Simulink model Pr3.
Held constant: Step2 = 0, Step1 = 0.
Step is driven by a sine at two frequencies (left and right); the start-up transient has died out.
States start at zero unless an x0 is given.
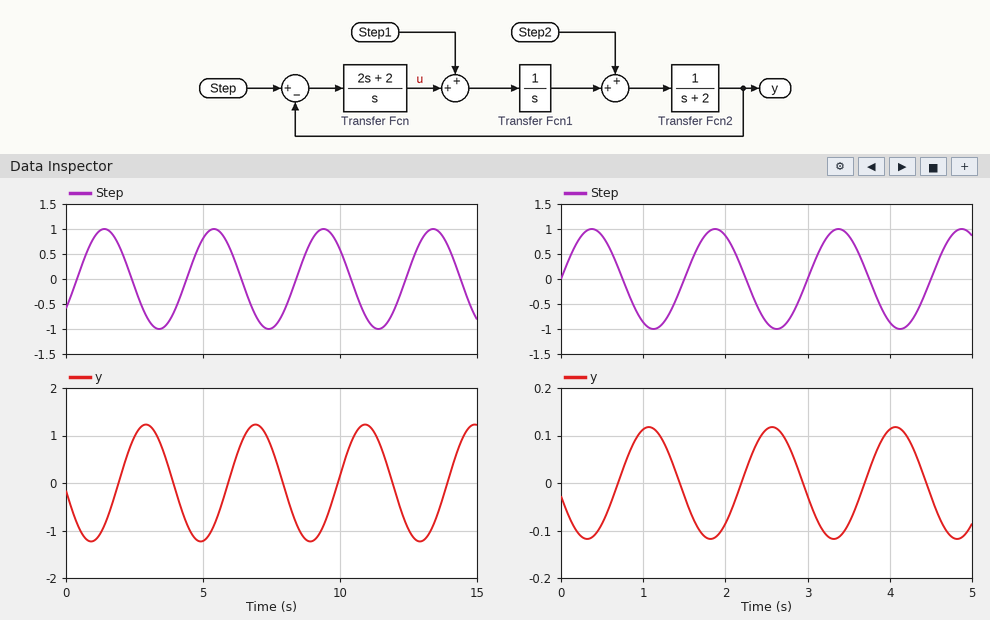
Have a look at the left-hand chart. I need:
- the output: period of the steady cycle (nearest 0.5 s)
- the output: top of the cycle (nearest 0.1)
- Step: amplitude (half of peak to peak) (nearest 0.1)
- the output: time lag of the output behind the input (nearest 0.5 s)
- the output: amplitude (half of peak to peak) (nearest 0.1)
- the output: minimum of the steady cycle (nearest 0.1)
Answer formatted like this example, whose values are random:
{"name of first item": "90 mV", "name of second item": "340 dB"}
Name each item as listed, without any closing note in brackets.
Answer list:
{"the output: period of the steady cycle": "4.0 s", "the output: top of the cycle": "1.2", "Step: amplitude (half of peak to peak)": "1.0", "the output: time lag of the output behind the input": "1.5 s", "the output: amplitude (half of peak to peak)": "1.2", "the output: minimum of the steady cycle": "-1.2"}
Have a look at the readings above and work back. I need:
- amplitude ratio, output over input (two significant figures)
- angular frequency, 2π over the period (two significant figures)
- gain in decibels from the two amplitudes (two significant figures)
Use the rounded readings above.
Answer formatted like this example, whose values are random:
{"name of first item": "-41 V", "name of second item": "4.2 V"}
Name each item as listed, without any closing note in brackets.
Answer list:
{"amplitude ratio, output over input": "1.2", "angular frequency, 2π over the period": "1.6 rad/s", "gain in decibels from the two amplitudes": "1.6 dB"}
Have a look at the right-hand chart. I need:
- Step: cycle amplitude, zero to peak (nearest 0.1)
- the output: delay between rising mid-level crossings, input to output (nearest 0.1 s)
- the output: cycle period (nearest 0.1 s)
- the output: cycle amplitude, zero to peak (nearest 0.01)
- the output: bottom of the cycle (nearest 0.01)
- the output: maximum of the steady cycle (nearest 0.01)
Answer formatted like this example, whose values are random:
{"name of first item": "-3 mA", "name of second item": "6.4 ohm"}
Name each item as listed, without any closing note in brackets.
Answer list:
{"Step: cycle amplitude, zero to peak": "1.0", "the output: delay between rising mid-level crossings, input to output": "0.7 s", "the output: cycle period": "1.5 s", "the output: cycle amplitude, zero to peak": "0.12", "the output: bottom of the cycle": "-0.12", "the output: maximum of the steady cycle": "0.12"}
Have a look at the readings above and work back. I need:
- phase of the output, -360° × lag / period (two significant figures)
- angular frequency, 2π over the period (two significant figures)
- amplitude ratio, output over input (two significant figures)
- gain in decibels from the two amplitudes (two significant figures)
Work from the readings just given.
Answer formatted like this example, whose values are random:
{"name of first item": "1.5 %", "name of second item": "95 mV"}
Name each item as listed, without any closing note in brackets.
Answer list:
{"phase of the output, -360° × lag / period": "-170°", "angular frequency, 2π over the period": "4.2 rad/s", "amplitude ratio, output over input": "0.12", "gain in decibels from the two amplitudes": "-18 dB"}
